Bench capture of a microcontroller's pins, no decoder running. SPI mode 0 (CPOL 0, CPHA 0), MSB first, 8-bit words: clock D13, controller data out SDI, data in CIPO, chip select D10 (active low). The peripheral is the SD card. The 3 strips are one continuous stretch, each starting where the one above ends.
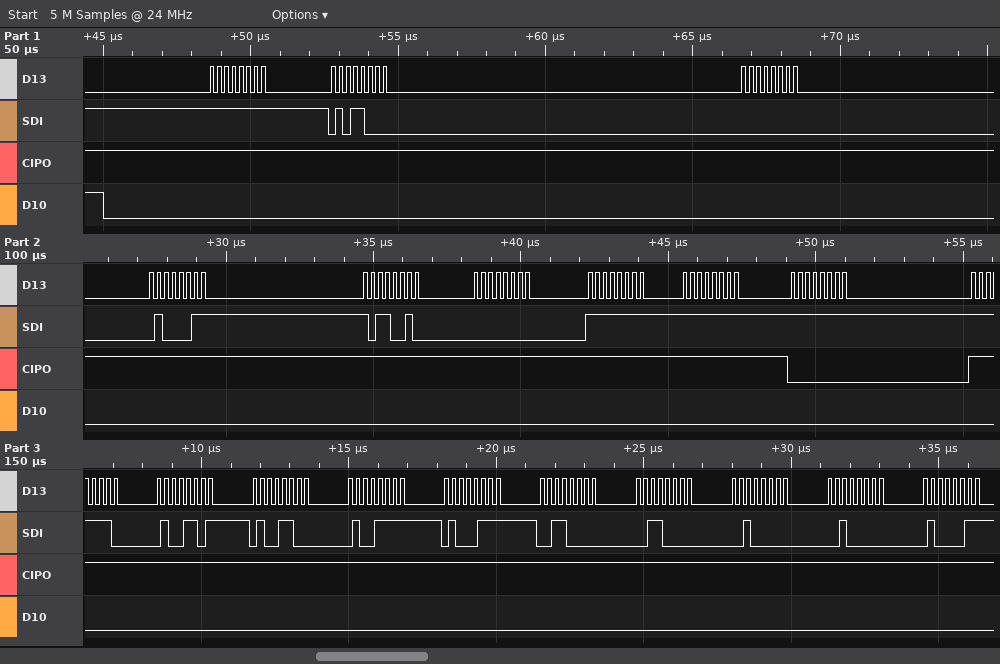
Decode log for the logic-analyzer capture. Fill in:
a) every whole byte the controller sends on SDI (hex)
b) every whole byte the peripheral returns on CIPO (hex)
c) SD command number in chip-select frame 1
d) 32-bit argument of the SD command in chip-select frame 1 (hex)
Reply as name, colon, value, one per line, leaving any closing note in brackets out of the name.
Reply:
every whole byte the controller sends on SDI: FF 58 00 43 B2 00 FF FF FF FE 4D 4C 4F 47 30 30 20 20 43
every whole byte the peripheral returns on CIPO: FF FF FF FF FF FF FF FF 00 FF FF FF FF FF FF FF FF FF FF
SD command number in chip-select frame 1: CMD24
32-bit argument of the SD command in chip-select frame 1: 0x0043B200
